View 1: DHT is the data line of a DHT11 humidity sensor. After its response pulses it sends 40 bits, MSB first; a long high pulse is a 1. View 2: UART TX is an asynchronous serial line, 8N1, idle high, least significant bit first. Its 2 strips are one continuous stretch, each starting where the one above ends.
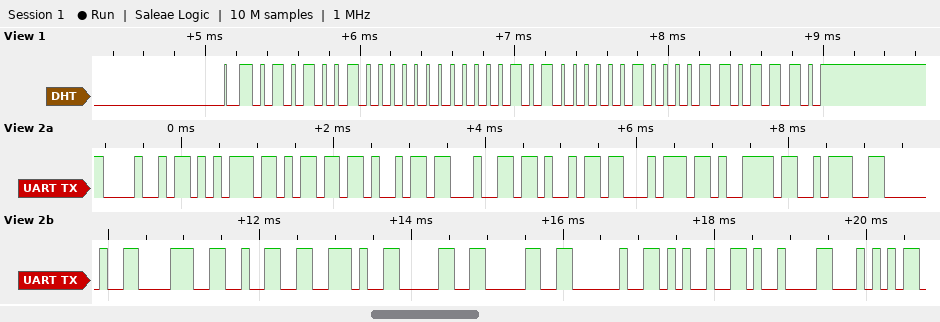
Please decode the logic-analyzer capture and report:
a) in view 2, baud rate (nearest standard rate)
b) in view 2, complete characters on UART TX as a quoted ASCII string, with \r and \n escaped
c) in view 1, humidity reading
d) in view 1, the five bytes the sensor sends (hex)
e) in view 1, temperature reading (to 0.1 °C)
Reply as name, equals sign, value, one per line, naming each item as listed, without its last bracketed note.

in view 2, baud rate = 9600 baud
in view 2, complete characters on UART TX as a quoted ASCII string, with \r and \n escaped = "Humidity: 82.00 %\tT"
in view 1, humidity reading = 82 %
in view 1, the five bytes the sensor sends = 52 00 14 08 6E
in view 1, temperature reading = 20.8 °C
